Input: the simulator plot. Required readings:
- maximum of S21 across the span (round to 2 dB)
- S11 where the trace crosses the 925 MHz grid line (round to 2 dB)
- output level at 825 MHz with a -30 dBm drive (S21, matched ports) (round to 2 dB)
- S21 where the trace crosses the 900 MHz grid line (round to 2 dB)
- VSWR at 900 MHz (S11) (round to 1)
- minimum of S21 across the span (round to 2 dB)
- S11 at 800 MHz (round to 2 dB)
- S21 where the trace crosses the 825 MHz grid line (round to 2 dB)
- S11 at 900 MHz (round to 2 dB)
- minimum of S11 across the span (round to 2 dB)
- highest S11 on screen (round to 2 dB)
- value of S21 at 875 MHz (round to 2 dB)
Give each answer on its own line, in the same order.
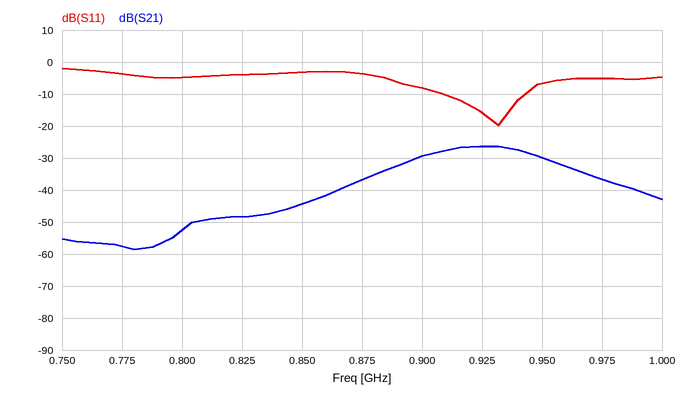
-26 dB
-16 dB
-78 dBm
-30 dB
2
-58 dB
-4 dB
-48 dB
-8 dB
-20 dB
-2 dB
-36 dB
